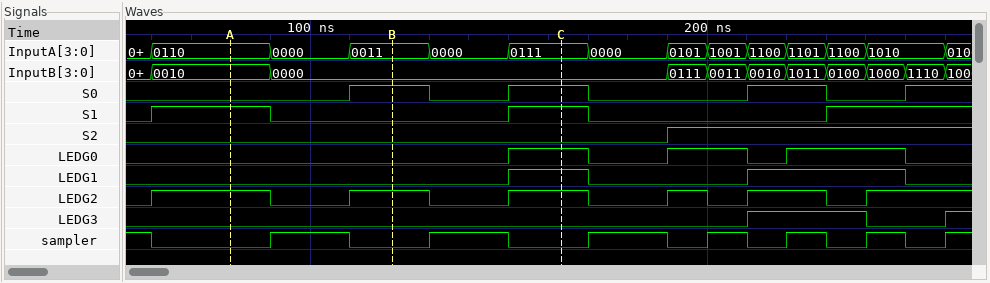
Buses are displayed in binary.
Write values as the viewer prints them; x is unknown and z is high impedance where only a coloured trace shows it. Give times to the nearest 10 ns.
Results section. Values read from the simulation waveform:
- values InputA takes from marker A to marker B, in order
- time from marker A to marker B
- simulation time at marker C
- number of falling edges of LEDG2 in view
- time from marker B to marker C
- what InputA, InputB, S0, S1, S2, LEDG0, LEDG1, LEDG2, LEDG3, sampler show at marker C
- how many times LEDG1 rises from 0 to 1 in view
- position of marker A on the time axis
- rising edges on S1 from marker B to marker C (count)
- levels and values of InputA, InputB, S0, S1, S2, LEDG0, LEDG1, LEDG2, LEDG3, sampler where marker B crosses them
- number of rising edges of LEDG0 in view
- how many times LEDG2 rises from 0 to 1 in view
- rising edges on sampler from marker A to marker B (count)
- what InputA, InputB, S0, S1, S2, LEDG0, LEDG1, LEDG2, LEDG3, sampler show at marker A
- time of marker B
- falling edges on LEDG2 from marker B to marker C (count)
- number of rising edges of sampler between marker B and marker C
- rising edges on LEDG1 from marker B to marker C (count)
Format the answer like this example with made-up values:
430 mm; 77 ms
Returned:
0110, 0000, 0011; 40 ns; 160 ns; 5; 40 ns; InputA=0111, InputB=0000, S0=1, S1=1, S2=0, LEDG0=1, LEDG1=1, LEDG2=1, LEDG3=0, sampler=0; 2; 80 ns; 1; InputA=0011, InputB=0000, S0=1, S1=0, S2=0, LEDG0=0, LEDG1=0, LEDG2=1, LEDG3=0, sampler=0; 3; 6; 1; InputA=0110, InputB=0010, S0=0, S1=1, S2=0, LEDG0=0, LEDG1=0, LEDG2=1, LEDG3=0, sampler=0; 120 ns; 1; 1; 1
